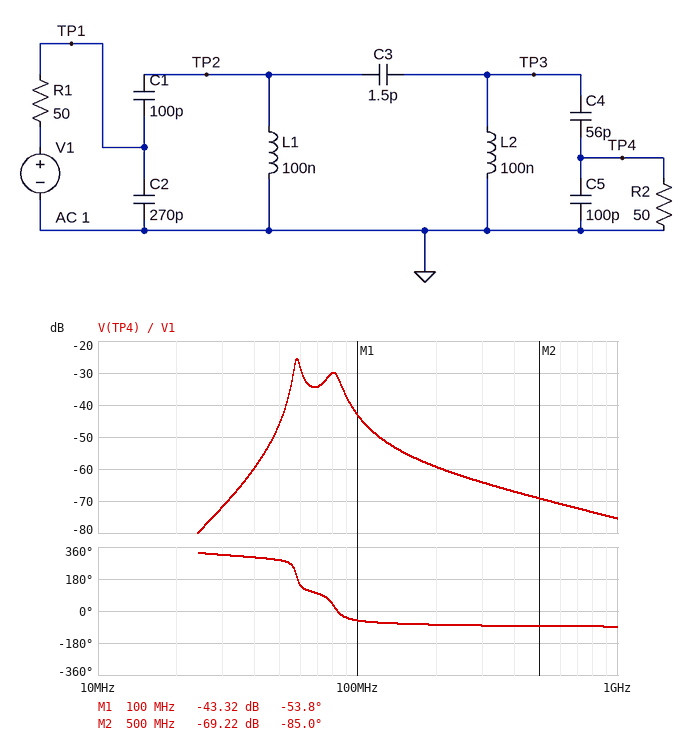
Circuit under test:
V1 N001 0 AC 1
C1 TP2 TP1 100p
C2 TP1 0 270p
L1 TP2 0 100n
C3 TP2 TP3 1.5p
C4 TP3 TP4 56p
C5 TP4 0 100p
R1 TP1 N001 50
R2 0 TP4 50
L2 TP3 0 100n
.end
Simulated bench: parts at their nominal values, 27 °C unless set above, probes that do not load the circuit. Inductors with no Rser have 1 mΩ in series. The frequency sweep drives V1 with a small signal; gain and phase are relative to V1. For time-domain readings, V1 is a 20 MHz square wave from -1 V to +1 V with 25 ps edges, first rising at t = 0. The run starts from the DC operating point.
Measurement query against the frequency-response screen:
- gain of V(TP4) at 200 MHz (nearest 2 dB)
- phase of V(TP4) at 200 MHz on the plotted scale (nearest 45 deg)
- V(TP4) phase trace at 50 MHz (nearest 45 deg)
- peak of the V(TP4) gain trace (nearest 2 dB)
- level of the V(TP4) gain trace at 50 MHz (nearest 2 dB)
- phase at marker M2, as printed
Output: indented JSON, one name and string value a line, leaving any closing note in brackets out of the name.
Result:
{
  "gain of V(TP4) at 200 MHz": "-60 dB",
  "phase of V(TP4) at 200 MHz on the plotted scale": "-90 deg",
  "V(TP4) phase trace at 50 MHz": "270 deg",
  "peak of the V(TP4) gain trace": "-26 dB",
  "level of the V(TP4) gain trace at 50 MHz": "-46 dB",
  "phase at marker M2, as printed": "-85.0 deg"
}
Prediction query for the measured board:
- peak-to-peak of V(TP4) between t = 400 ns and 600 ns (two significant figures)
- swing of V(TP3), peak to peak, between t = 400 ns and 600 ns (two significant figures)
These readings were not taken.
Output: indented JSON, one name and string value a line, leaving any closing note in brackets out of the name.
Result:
{
  "peak-to-peak of V(TP4) between t = 400 ns and 600 ns": "35 mV",
  "swing of V(TP3), peak to peak, between t = 400 ns and 600 ns": "100 mV"
}
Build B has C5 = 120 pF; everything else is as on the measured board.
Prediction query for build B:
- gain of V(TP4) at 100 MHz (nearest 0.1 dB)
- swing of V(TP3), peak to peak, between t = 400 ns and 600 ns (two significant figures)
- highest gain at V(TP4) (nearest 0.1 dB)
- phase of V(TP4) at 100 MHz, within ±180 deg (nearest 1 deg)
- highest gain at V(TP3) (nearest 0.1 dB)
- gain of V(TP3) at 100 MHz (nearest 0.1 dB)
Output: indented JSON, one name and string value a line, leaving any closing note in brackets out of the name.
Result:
{
  "gain of V(TP4) at 100 MHz": "-45.4 dB",
  "swing of V(TP3), peak to peak, between t = 400 ns and 600 ns": "110 mV",
  "highest gain at V(TP4)": "-26.0 dB",
  "phase of V(TP4) at 100 MHz, within ±180 deg": "-60 deg",
  "highest gain at V(TP3)": "-15.7 dB",
  "gain of V(TP3) at 100 MHz": "-35.3 dB"
}
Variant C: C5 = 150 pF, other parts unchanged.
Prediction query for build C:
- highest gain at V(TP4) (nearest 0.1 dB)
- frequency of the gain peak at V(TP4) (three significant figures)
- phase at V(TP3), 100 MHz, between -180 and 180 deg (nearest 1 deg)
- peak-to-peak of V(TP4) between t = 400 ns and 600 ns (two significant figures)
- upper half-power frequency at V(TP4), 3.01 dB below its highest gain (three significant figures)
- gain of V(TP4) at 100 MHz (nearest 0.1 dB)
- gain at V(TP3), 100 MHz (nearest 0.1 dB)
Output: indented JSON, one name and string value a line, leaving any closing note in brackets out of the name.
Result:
{
  "highest gain at V(TP4)": "-26.5 dB",
  "frequency of the gain peak at V(TP4)": "76.7 MHz",
  "phase at V(TP3), 100 MHz, between -180 and 180 deg": "-75 deg",
  "peak-to-peak of V(TP4) between t = 400 ns and 600 ns": "30 mV",
  "upper half-power frequency at V(TP4), 3.01 dB below its highest gain": "79.2 MHz",
  "gain of V(TP4) at 100 MHz": "-47.9 dB",
  "gain at V(TP3), 100 MHz": "-36.5 dB"
}
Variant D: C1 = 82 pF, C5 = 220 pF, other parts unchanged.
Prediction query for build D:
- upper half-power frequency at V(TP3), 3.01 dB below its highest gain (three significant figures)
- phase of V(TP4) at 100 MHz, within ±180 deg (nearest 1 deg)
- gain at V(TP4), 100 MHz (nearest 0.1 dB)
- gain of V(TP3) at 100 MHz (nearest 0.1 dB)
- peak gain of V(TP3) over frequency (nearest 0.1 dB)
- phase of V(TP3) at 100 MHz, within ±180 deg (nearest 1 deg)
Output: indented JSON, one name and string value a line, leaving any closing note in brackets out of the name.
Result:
{
  "upper half-power frequency at V(TP3), 3.01 dB below its highest gain": "75.2 MHz",
  "phase of V(TP4) at 100 MHz, within ±180 deg": "-72 deg",
  "gain at V(TP4), 100 MHz": "-51.3 dB",
  "gain of V(TP3) at 100 MHz": "-37.4 dB",
  "peak gain of V(TP3) over frequency": "-6.7 dB",
  "phase of V(TP3) at 100 MHz, within ±180 deg": "-79 deg"
}
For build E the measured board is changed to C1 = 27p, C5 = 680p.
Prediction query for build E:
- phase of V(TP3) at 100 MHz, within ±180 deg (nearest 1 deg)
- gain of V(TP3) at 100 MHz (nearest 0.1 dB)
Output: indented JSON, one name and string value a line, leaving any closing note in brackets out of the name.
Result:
{
  "phase of V(TP3) at 100 MHz, within ±180 deg": "-62 deg",
  "gain of V(TP3) at 100 MHz": "-13.3 dB"
}
